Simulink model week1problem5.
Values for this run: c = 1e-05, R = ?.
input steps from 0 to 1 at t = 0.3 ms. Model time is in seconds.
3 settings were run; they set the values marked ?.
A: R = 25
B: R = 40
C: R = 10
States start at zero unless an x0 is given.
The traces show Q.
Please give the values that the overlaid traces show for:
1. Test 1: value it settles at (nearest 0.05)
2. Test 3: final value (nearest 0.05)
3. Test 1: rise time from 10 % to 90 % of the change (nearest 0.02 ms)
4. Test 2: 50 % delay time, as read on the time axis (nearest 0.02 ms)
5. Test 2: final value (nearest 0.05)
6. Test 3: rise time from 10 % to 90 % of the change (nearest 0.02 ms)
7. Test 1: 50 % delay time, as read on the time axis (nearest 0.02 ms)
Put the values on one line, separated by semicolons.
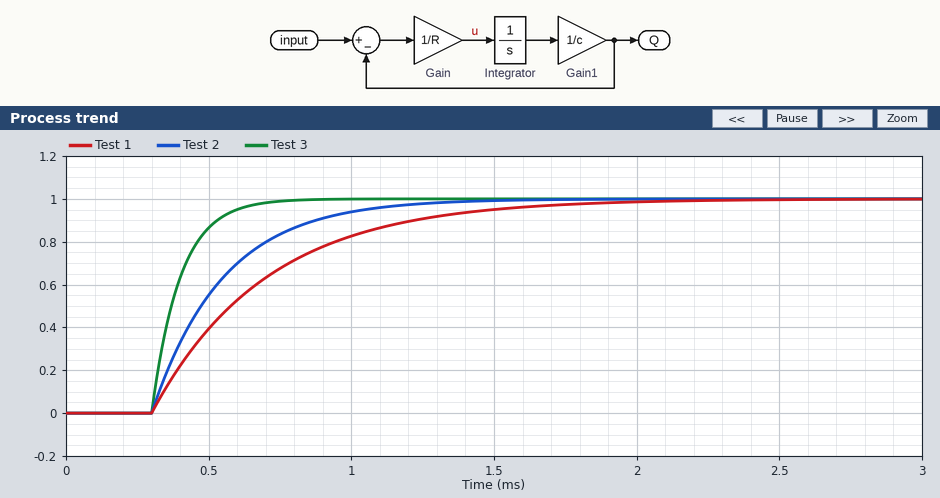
1.00; 1.00; 0.88 ms; 0.48 ms; 1.00; 0.22 ms; 0.58 ms
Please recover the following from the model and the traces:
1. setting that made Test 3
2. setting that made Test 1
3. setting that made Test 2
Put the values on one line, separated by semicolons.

C; B; A
